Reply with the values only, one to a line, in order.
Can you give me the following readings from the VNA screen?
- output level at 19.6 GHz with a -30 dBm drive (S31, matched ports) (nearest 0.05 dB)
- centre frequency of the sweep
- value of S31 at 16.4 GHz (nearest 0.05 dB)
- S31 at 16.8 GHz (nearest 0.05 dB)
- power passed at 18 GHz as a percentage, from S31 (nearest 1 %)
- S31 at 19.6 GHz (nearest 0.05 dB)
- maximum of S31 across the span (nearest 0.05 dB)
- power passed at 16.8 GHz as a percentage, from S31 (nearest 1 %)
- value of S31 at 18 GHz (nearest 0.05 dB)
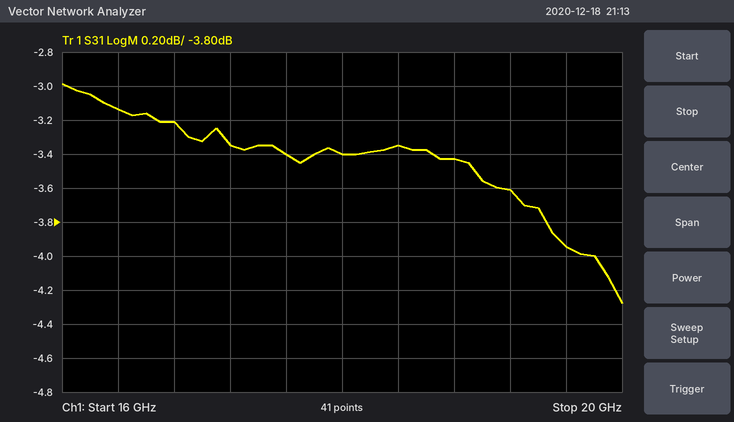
-33.95 dBm
18 GHz
-3.15 dB
-3.20 dB
46 %
-3.95 dB
-3.00 dB
48 %
-3.40 dB
